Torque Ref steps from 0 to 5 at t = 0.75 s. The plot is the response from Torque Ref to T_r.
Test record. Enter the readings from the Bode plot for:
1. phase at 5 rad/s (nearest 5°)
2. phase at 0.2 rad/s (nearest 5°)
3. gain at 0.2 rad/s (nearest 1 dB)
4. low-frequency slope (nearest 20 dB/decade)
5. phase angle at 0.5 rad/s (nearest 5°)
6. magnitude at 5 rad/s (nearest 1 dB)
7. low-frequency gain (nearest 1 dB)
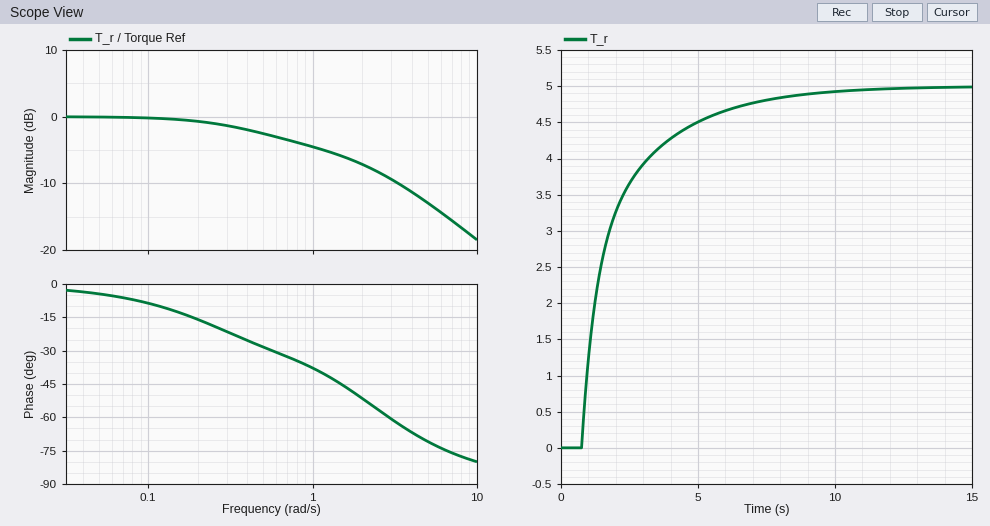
-70°
-15°
-1 dB
0 dB/decade
-30°
-13 dB
0 dB
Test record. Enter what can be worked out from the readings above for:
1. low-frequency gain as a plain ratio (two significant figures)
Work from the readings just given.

1.0
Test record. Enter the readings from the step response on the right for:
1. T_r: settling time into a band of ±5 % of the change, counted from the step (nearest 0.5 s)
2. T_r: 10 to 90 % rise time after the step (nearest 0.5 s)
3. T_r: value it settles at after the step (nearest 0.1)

6.0 s
4.0 s
5.0
